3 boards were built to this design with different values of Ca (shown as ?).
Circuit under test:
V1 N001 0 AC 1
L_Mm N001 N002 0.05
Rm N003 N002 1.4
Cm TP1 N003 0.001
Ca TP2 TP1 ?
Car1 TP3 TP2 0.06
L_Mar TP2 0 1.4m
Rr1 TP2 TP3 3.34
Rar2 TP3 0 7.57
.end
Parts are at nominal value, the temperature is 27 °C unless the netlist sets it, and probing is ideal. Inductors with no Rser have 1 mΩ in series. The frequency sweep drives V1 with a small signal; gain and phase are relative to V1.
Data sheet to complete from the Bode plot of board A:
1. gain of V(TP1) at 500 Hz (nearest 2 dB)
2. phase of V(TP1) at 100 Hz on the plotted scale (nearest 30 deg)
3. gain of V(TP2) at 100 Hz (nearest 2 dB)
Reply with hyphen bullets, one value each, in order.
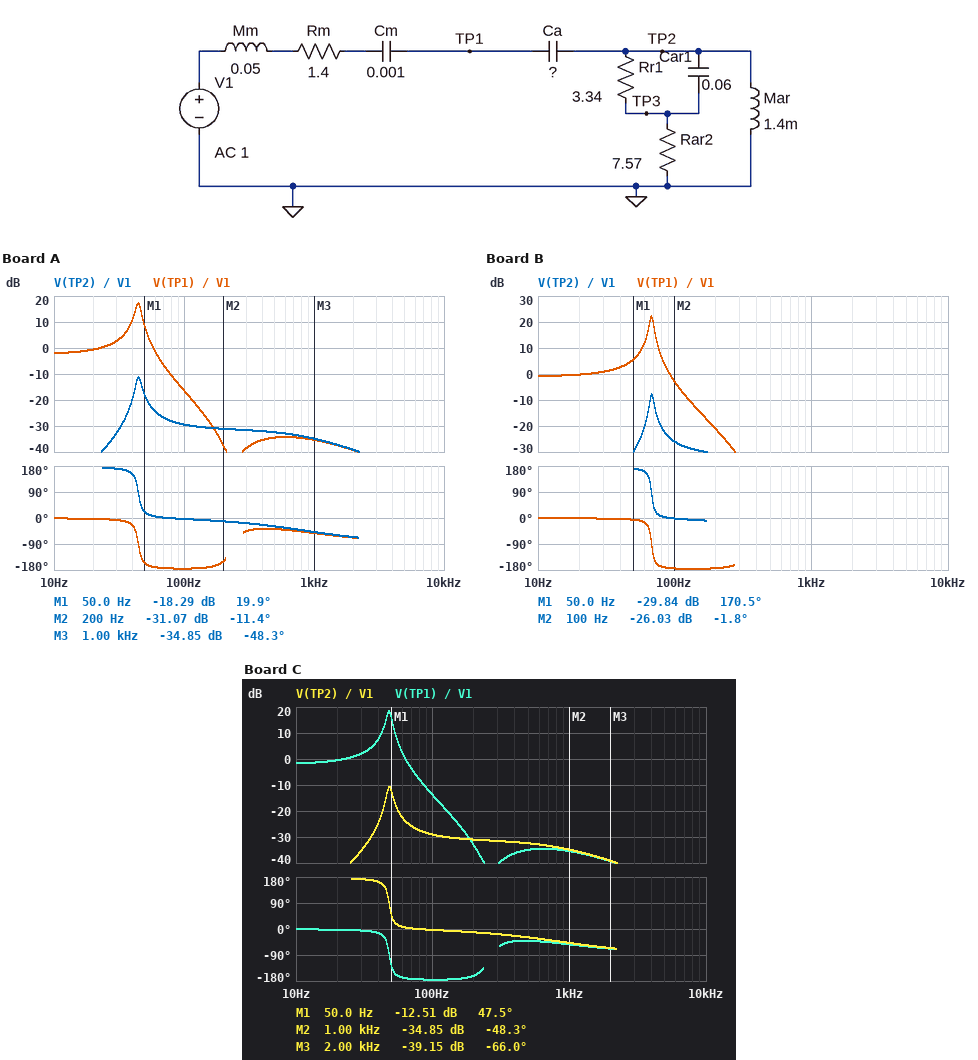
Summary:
- -34 dB
- -180 deg
- -30 dB
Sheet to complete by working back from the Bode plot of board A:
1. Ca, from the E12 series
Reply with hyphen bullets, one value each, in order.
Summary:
- 330 µF
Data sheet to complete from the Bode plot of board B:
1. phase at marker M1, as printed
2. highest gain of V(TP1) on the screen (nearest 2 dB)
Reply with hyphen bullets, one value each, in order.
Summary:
- 170.5 deg
- 22 dB
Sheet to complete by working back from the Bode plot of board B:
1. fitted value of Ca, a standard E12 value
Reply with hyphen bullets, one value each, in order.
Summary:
- 120 µF
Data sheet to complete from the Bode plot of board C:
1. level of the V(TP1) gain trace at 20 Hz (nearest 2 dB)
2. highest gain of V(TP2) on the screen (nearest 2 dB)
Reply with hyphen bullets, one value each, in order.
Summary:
- 0 dB
- -10 dB
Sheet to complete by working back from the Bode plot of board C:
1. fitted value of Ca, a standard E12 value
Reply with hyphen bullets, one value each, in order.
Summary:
- 270 µF
